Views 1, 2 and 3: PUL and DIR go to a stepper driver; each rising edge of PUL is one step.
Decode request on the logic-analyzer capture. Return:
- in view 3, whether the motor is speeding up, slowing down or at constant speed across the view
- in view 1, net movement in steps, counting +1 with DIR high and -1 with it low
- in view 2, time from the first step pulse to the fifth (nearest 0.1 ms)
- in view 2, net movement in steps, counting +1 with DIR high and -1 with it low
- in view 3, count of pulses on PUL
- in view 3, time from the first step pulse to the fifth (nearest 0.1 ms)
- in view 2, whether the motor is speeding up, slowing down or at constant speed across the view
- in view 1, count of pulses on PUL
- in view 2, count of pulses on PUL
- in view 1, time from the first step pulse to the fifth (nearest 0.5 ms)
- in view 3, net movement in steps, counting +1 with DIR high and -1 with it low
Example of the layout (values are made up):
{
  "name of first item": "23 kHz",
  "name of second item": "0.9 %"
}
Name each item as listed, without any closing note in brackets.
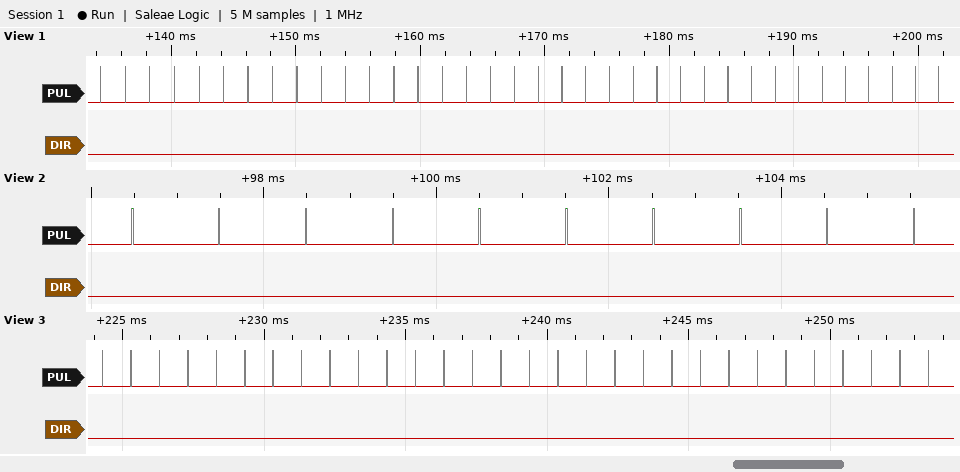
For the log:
{
  "in view 3, whether the motor is speeding up, slowing down or at constant speed across the view": "constant speed",
  "in view 1, net movement in steps, counting +1 with DIR high and -1 with it low": "-36",
  "in view 2, time from the first step pulse to the fifth": "4.0 ms",
  "in view 2, net movement in steps, counting +1 with DIR high and -1 with it low": "-10",
  "in view 3, count of pulses on PUL": "30",
  "in view 3, time from the first step pulse to the fifth": "4.0 ms",
  "in view 2, whether the motor is speeding up, slowing down or at constant speed across the view": "constant speed",
  "in view 1, count of pulses on PUL": "36",
  "in view 2, count of pulses on PUL": "10",
  "in view 1, time from the first step pulse to the fifth": "8.0 ms",
  "in view 3, net movement in steps, counting +1 with DIR high and -1 with it low": "-30"
}
